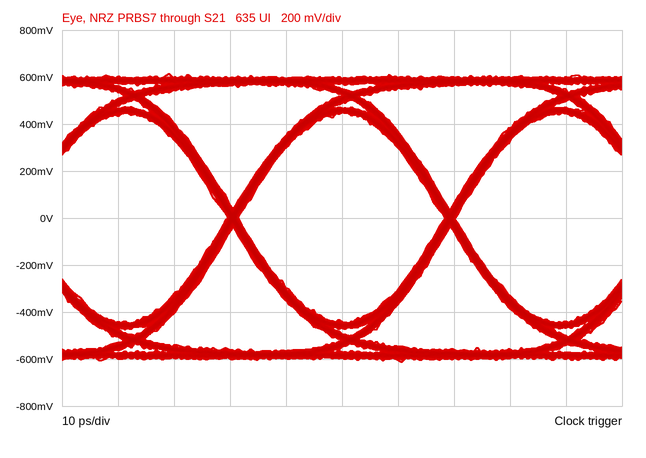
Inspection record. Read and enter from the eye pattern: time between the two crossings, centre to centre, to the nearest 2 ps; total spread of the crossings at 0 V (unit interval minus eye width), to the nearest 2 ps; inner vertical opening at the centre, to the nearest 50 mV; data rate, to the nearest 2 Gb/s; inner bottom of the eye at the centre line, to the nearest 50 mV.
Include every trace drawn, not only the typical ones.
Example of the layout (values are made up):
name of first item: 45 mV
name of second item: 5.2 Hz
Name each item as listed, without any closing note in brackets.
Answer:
time between the two crossings, centre to centre, to the nearest 2 ps: 38 ps
total spread of the crossings at 0 V (unit interval minus eye width), to the nearest 2 ps: 2 ps
inner vertical opening at the centre, to the nearest 50 mV: 900 mV
data rate, to the nearest 2 Gb/s: 26 Gb/s
inner bottom of the eye at the centre line, to the nearest 50 mV: -450 mV
